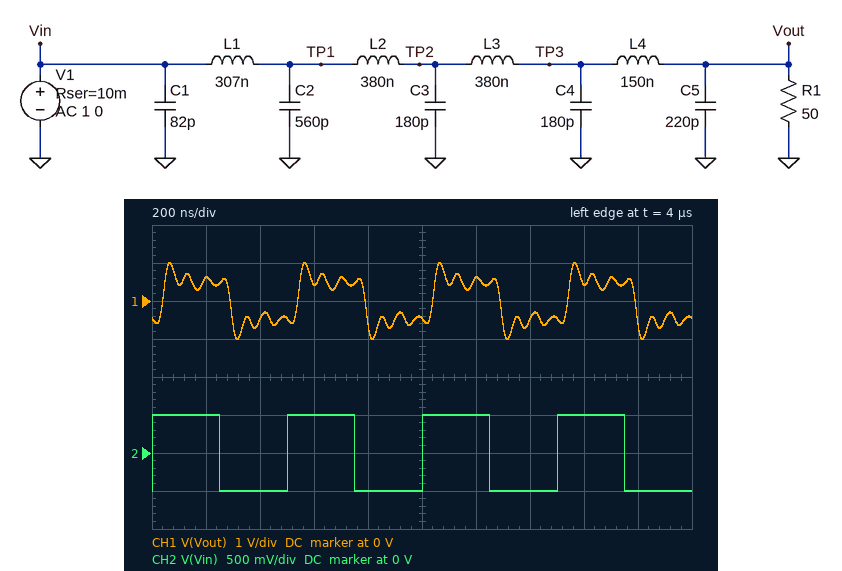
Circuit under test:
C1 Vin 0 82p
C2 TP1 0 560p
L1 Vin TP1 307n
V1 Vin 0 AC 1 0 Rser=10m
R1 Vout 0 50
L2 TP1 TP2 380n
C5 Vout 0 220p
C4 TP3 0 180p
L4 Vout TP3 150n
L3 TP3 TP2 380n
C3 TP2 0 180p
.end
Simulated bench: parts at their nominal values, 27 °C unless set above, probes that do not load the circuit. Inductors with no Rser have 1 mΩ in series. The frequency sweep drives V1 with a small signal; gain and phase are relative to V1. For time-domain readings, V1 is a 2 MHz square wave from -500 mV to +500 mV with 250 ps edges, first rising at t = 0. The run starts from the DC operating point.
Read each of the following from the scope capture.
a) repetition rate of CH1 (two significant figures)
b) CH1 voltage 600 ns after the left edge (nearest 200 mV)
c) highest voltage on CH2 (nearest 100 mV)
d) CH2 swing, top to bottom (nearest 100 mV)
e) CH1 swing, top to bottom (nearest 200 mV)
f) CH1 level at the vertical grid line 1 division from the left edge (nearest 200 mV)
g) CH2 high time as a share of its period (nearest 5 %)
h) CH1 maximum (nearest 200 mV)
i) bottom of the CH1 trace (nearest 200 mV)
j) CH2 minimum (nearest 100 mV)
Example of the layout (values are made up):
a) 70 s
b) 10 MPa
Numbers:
a) 2.0 MHz
b) 400 mV
c) 500 mV
d) 1.0 V
e) 2.0 V
f) 600 mV
g) 50 %
h) 1.0 V
i) -1.0 V
j) -500 mV
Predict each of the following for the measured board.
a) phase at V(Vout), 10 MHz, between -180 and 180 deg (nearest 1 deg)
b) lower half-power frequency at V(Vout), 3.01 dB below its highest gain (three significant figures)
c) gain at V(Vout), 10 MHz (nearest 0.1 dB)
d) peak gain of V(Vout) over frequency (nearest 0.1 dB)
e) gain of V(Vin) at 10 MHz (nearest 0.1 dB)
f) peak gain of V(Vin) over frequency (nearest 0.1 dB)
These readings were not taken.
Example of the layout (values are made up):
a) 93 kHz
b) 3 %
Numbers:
a) -142 deg
b) 13.2 MHz
c) 1.9 dB
d) 8.8 dB
e) 0 dB
f) 0 dB
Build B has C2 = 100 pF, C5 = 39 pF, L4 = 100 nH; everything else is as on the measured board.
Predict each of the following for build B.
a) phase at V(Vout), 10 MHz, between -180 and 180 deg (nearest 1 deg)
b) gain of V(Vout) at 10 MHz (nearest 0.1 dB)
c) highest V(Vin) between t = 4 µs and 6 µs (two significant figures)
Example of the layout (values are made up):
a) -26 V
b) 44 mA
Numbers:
a) -105 deg
b) -0.2 dB
c) 500 mV
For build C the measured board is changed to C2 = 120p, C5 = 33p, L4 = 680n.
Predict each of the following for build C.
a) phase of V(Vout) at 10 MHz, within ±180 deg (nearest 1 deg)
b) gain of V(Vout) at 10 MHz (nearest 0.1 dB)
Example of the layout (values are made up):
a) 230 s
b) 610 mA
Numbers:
a) -106 deg
b) 1.0 dB
